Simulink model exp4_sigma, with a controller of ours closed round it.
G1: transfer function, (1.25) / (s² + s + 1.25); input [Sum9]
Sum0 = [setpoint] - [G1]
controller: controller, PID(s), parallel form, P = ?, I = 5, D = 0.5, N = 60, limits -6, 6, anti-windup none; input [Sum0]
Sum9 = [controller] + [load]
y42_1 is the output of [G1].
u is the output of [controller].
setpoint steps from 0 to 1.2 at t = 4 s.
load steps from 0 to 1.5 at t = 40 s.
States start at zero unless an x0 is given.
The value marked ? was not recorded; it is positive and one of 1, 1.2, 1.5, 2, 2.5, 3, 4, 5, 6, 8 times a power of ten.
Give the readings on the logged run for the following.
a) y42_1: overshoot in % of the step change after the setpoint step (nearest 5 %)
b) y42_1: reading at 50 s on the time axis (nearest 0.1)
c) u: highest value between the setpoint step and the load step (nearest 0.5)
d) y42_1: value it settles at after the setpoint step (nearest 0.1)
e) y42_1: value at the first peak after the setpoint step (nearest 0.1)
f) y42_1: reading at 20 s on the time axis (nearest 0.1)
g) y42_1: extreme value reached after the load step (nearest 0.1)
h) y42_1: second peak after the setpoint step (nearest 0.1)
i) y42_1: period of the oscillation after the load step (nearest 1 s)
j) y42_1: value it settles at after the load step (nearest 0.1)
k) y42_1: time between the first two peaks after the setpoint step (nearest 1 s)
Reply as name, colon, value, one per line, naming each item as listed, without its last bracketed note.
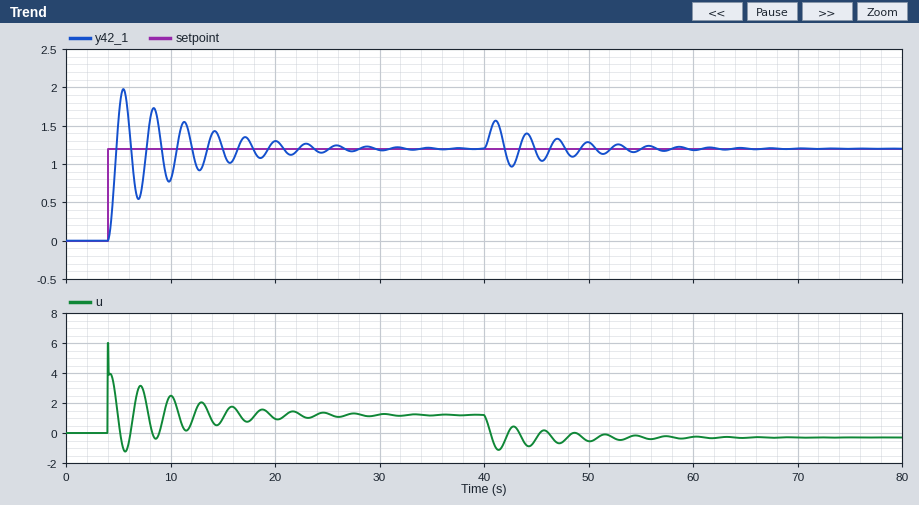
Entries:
y42_1: overshoot in % of the step change after the setpoint step: 65 %
y42_1: reading at 50 s on the time axis: 1.3
u: highest value between the setpoint step and the load step: 6.0
y42_1: value it settles at after the setpoint step: 1.2
y42_1: value at the first peak after the setpoint step: 2.0
y42_1: reading at 20 s on the time axis: 1.3
y42_1: extreme value reached after the load step: 1.6
y42_1: second peak after the setpoint step: 1.7
y42_1: period of the oscillation after the load step: 3 s
y42_1: value it settles at after the load step: 1.2
y42_1: time between the first two peaks after the setpoint step: 3 s
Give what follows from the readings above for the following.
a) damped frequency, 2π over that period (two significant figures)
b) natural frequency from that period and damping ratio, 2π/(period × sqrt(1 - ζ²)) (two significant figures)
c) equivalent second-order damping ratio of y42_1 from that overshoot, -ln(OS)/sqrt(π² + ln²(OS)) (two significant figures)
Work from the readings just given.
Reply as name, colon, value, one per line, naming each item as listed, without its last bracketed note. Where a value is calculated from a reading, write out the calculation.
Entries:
damped frequency, 2π over that period: 2π / 3 = 2.1 rad/s
natural frequency from that period and damping ratio, 2π/(period × sqrt(1 - ζ²)): 2π / (3 × sqrt(1 - 0.14²)) = 2.1 rad/s
equivalent second-order damping ratio of y42_1 from that overshoot, -ln(OS)/sqrt(π² + ln²(OS)): ln(0.65) = -0.431; 0.431 / sqrt(9.870 + 0.186) = 0.14
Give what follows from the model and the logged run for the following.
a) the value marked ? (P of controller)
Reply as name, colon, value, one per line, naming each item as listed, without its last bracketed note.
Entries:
the value marked ?: 3
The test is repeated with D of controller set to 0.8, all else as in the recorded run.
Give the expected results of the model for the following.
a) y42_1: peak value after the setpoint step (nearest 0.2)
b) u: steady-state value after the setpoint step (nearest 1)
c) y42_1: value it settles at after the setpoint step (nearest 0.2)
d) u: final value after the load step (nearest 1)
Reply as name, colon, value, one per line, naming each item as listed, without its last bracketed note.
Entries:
y42_1: peak value after the setpoint step: 1.8
u: steady-state value after the setpoint step: 1
y42_1: value it settles at after the setpoint step: 1.2
u: final value after the load step: 0
